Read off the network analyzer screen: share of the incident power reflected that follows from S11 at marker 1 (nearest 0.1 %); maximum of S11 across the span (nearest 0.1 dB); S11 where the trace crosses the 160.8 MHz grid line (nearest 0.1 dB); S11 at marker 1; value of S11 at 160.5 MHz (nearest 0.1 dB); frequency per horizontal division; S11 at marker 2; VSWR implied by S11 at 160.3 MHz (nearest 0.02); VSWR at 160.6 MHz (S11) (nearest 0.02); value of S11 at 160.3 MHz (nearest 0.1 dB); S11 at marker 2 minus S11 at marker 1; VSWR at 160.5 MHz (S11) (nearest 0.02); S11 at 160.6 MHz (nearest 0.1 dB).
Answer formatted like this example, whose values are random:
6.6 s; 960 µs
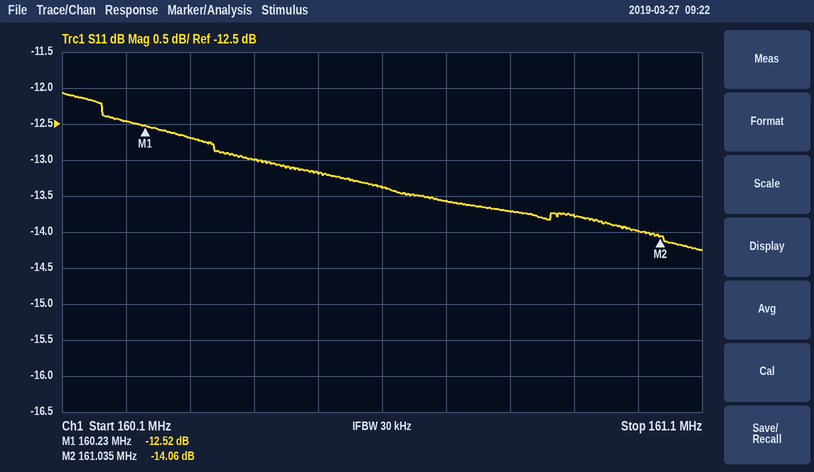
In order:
5.6 %; -12.1 dB; -13.7 dB; -12.52 dB; -13.2 dB; 100 kHz; -14.06 dB; 1.60; 1.54; -12.7 dB; -1.54 dB; 1.56; -13.4 dB
